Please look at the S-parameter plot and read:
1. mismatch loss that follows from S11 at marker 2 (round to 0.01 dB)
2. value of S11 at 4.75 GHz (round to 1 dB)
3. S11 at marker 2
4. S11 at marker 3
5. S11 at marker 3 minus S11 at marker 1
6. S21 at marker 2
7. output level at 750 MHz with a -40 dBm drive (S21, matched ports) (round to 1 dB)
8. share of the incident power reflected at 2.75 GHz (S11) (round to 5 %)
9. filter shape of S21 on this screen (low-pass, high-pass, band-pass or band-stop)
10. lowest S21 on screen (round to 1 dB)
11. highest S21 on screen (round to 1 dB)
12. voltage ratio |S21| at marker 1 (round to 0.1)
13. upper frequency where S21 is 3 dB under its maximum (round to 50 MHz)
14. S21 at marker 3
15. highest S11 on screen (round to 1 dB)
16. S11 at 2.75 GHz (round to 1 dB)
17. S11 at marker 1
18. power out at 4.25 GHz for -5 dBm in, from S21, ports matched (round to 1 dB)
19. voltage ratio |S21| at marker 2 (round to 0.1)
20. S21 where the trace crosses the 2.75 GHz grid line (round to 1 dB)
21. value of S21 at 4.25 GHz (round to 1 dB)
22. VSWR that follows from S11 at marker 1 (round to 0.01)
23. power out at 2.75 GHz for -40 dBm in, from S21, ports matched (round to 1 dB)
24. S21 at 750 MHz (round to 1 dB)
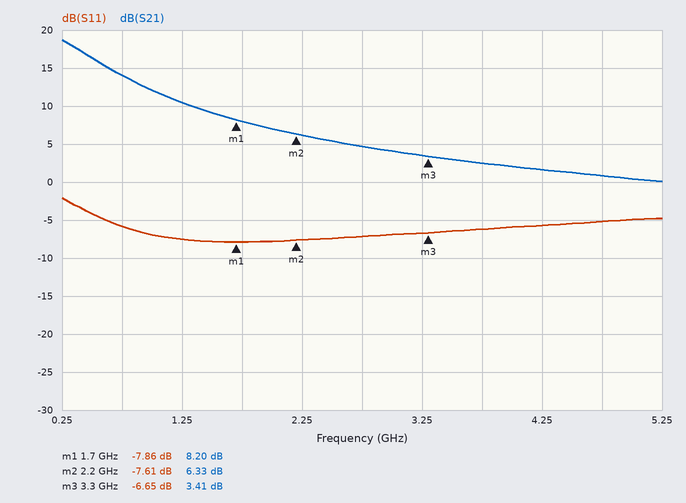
0.83 dB
-5 dB
-7.61 dB
-6.65 dB
1.21 dB
6.33 dB
-26 dBm
20 %
low-pass
0 dB
19 dB
2.6
550 MHz
3.41 dB
-2 dB
-7 dB
-7.86 dB
-3 dBm
2.1
5 dB
2 dB
2.36
-35 dBm
14 dB
